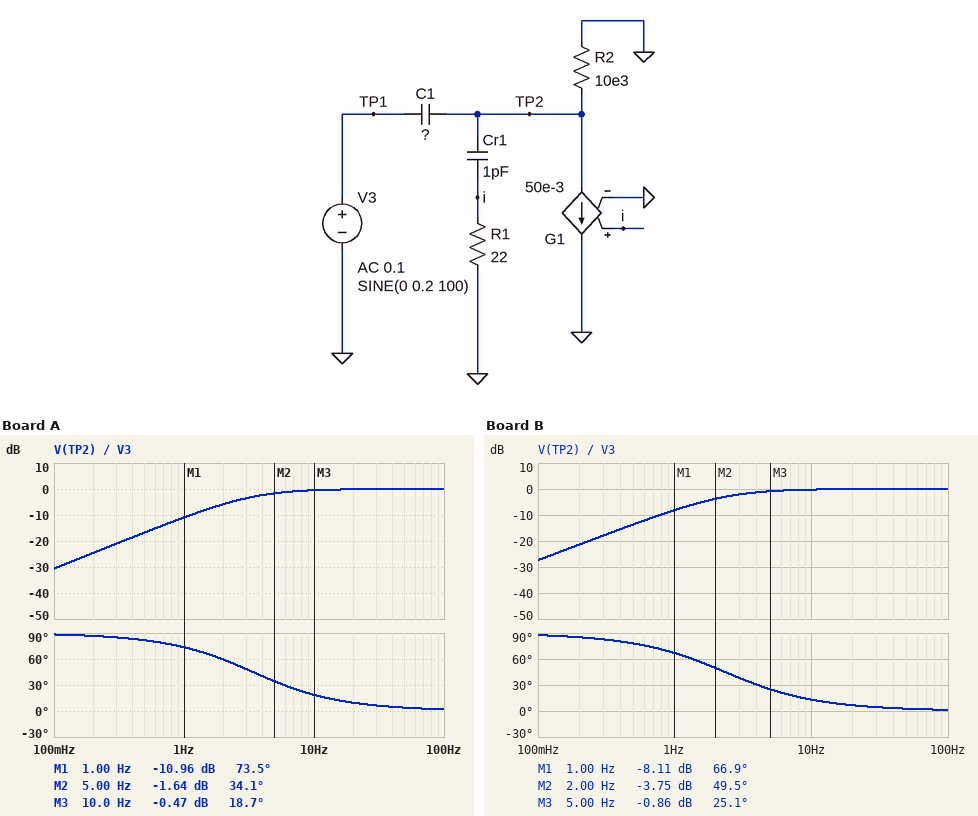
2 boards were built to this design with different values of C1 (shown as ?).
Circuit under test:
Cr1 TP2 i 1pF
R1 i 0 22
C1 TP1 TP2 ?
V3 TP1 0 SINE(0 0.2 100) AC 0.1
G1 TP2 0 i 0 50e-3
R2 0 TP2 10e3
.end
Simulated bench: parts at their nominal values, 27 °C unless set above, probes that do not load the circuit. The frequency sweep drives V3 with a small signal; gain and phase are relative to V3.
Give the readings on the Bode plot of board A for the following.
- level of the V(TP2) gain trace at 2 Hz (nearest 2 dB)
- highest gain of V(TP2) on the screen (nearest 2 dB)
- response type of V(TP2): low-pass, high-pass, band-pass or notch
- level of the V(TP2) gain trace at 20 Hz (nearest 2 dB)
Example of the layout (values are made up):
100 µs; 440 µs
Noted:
-6 dB; 0 dB; high-pass; 0 dB
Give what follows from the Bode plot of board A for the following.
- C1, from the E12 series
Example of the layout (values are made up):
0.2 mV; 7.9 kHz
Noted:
4.7 µF
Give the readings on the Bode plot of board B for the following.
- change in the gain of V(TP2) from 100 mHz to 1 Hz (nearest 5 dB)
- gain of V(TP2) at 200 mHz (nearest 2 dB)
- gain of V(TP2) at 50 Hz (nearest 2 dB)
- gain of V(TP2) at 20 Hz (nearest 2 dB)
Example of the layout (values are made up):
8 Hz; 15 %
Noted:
20 dB; -22 dB; 0 dB; 0 dB
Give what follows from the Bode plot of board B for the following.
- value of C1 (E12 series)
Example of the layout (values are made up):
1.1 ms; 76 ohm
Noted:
6.8 µF
